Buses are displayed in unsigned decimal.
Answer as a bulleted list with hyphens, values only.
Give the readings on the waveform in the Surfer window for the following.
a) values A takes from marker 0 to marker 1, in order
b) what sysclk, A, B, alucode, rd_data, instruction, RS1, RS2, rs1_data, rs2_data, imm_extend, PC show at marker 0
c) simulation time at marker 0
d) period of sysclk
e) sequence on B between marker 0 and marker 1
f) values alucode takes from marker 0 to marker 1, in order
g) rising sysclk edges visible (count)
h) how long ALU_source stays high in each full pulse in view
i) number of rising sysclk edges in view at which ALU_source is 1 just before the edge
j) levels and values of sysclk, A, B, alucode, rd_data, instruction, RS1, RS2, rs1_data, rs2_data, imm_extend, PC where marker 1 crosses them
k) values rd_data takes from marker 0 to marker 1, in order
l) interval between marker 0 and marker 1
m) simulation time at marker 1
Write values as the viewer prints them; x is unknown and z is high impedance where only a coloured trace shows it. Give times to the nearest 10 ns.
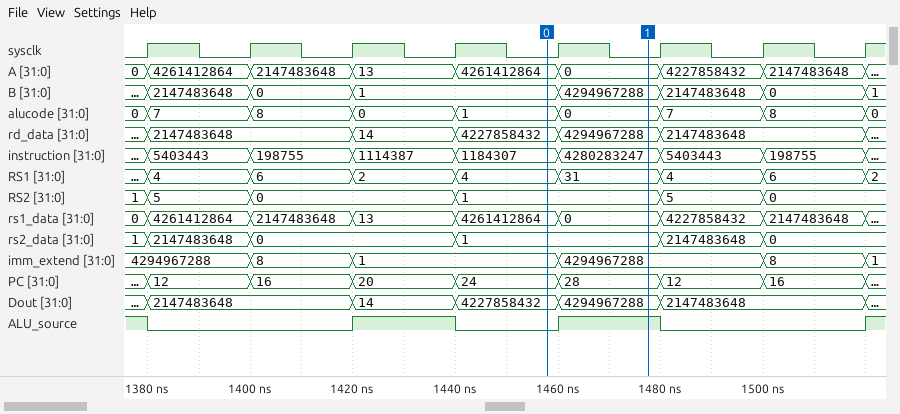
- 4261412864, 0
- sysclk=0, A=4261412864, B=1, alucode=1, rd_data=4227858432, instruction=1184307, RS1=4, RS2=1, rs1_data=4261412864, rs2_data=1, imm_extend=1, PC=24
- 1460 ns
- 20 ns
- 1, 4294967288
- 1, 0
- 8
- 20 ns, 20 ns
- 3
- sysclk=0, A=0, B=4294967288, alucode=0, rd_data=4294967288, instruction=4280283247, RS1=31, RS2=1, rs1_data=0, rs2_data=1, imm_extend=4294967288, PC=28
- 4227858432, 4294967288
- 20 ns
- 1480 ns
